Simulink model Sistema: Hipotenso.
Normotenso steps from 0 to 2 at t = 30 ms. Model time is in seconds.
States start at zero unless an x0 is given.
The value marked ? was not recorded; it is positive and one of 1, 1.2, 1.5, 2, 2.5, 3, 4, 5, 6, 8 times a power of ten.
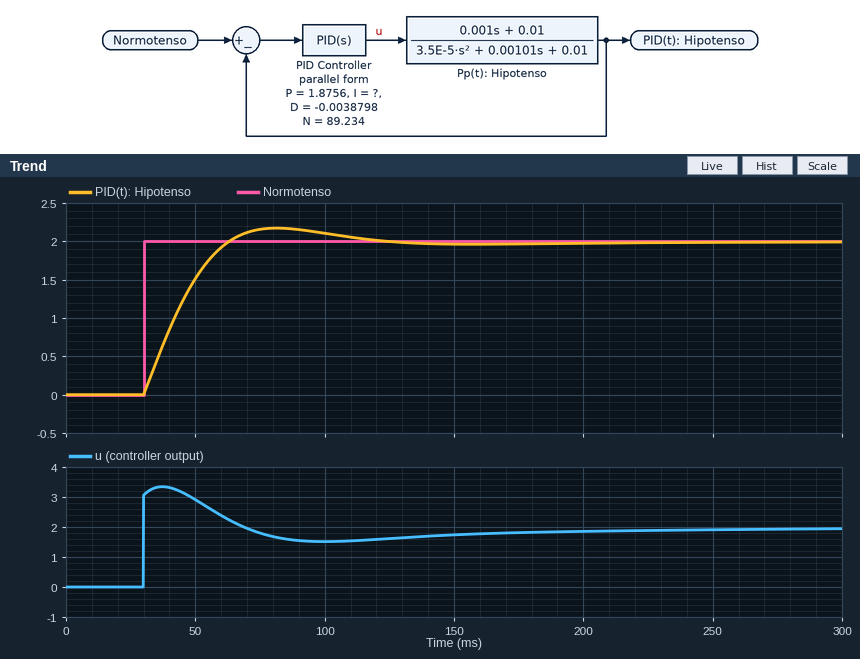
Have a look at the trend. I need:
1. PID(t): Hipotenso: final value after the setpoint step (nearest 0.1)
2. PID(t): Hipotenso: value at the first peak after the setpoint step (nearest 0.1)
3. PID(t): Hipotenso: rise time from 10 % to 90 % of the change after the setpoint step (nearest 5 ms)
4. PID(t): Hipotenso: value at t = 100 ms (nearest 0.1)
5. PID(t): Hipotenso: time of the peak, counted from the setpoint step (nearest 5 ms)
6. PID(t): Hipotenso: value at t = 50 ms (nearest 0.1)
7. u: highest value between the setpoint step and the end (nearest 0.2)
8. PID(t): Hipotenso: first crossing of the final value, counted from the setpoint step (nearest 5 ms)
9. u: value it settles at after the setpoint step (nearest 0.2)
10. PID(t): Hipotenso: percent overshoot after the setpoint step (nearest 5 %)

2.0
2.2
25 ms
2.1
50 ms
1.5
3.4
35 ms
2.0
10 %
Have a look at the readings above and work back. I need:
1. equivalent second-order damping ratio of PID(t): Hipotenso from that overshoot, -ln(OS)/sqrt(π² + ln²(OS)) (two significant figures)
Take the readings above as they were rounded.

0.59
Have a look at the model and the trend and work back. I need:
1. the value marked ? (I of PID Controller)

80
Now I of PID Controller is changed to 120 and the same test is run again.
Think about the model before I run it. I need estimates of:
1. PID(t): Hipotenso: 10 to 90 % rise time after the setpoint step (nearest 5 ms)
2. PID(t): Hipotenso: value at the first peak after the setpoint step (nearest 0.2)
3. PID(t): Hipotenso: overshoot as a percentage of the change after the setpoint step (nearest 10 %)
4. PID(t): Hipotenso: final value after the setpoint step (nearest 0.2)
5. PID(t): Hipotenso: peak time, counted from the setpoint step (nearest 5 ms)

20 ms
2.4
20 %
2.0
45 ms
